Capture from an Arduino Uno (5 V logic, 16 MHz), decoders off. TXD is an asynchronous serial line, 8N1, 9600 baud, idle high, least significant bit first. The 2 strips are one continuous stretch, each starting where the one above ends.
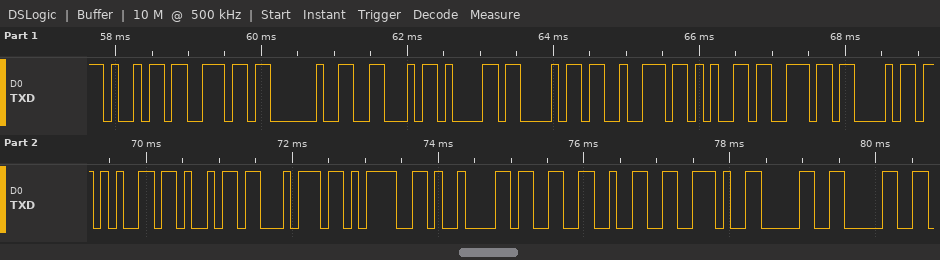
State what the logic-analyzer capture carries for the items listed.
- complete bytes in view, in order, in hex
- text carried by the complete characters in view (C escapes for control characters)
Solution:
69 6E 20 46 61 68 72 65 6E 68 65 69 74 3D 09 33 32 2E 30 30
"in Fahrenheit=\t32.00"
